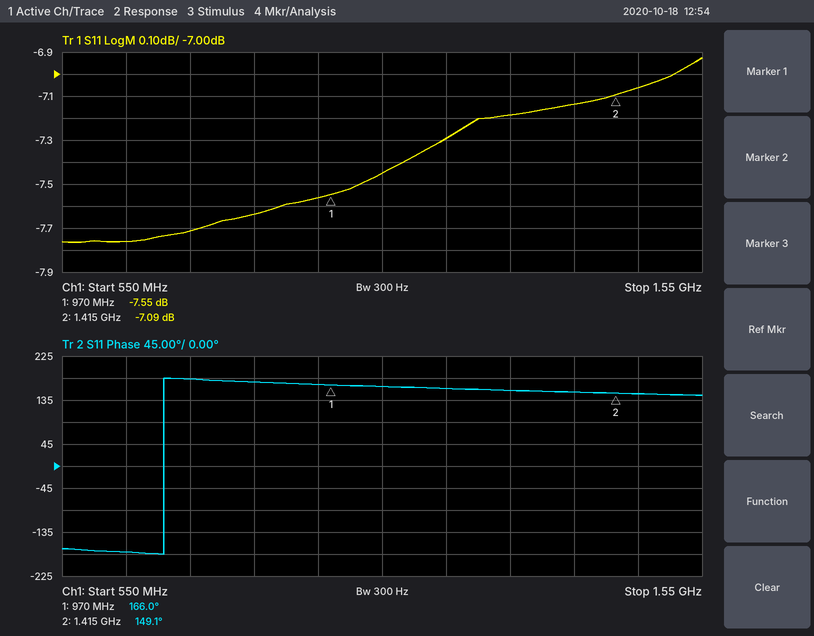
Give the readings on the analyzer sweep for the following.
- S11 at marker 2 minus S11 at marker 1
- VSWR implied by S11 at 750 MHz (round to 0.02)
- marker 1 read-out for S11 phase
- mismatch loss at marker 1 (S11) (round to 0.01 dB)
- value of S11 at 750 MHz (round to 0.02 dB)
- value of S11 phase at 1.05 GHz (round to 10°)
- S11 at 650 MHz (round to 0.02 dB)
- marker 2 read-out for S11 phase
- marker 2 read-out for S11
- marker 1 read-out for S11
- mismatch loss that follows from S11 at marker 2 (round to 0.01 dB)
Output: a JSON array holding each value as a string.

["0.46 dB", "2.40", "166.0°", "0.84 dB", "-7.72 dB", "160°", "-7.76 dB", "149.1°", "-7.09 dB", "-7.55 dB", "0.94 dB"]
